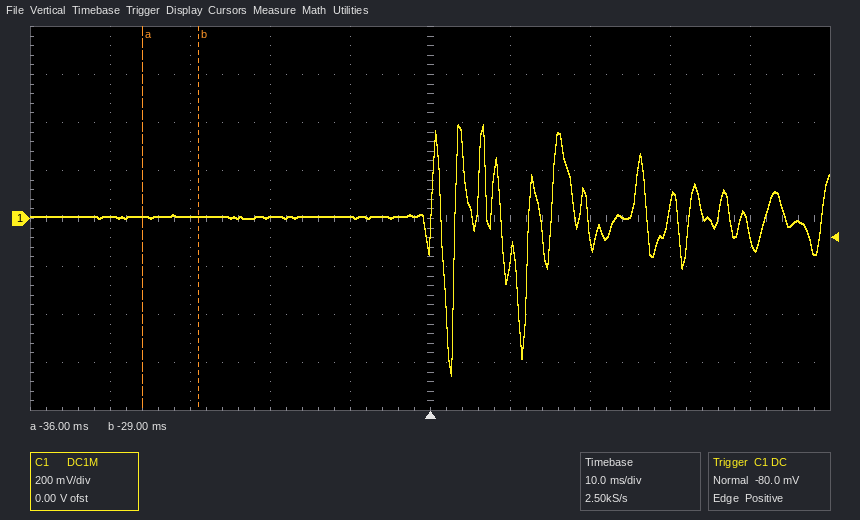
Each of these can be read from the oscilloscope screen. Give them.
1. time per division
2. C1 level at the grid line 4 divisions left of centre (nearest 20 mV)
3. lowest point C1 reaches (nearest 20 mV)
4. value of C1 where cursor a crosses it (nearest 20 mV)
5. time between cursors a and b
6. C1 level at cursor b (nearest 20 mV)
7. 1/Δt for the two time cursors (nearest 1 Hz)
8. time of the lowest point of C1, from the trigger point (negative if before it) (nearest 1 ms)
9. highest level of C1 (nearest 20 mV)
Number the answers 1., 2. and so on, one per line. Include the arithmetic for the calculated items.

1. 10 ms
2. 0 mV
3. -660 mV
4. 0 mV
5. -29 ms − (-36 ms) = 7 ms
6. 0 mV
7. 1 / 7 ms ≈ 143 Hz
8. +3 ms
9. 400 mV
